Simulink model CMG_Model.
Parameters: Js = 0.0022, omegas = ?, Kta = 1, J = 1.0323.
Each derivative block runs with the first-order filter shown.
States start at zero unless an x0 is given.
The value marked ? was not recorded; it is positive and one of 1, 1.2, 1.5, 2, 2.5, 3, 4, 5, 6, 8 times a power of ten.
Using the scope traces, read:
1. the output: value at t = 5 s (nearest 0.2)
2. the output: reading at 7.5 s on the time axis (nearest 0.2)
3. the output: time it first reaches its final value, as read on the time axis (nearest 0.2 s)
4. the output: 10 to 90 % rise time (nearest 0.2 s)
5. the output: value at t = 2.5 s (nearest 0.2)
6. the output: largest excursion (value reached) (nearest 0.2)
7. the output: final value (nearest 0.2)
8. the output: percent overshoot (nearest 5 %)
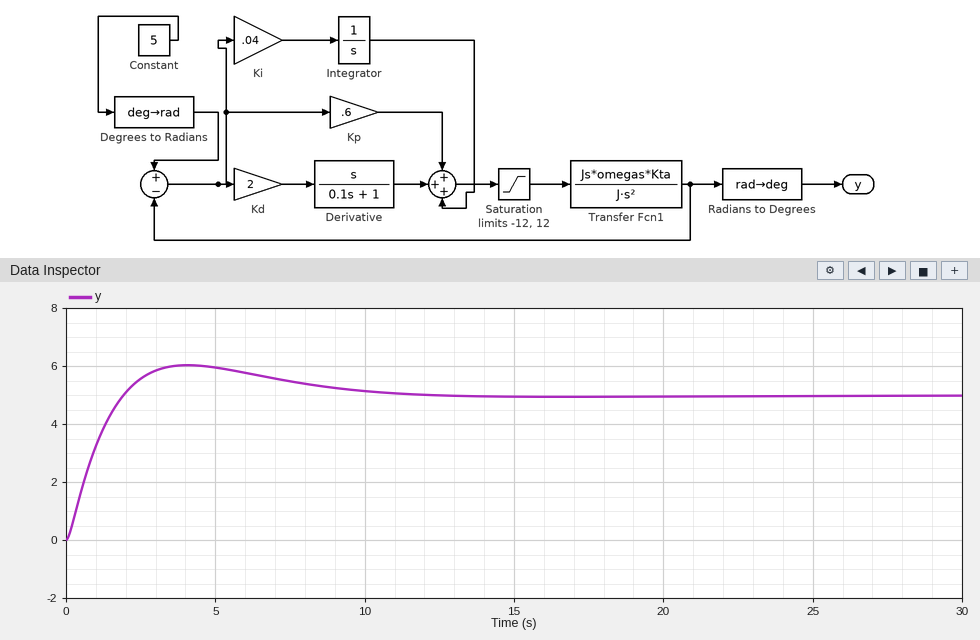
6.0
5.4
2.0 s
1.4 s
5.6
6.0
5.0
20 %
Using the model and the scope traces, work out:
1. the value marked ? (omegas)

200
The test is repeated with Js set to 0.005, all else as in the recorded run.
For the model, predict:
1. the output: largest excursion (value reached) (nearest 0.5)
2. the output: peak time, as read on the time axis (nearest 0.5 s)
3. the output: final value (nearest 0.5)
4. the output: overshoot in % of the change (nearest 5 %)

5.5
2.0 s
5.0
10 %
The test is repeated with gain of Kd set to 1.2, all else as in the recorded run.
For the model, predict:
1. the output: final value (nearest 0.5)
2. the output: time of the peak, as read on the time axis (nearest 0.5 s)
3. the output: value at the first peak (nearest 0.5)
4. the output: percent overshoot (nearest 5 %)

5.0
4.5 s
7.0
35 %
